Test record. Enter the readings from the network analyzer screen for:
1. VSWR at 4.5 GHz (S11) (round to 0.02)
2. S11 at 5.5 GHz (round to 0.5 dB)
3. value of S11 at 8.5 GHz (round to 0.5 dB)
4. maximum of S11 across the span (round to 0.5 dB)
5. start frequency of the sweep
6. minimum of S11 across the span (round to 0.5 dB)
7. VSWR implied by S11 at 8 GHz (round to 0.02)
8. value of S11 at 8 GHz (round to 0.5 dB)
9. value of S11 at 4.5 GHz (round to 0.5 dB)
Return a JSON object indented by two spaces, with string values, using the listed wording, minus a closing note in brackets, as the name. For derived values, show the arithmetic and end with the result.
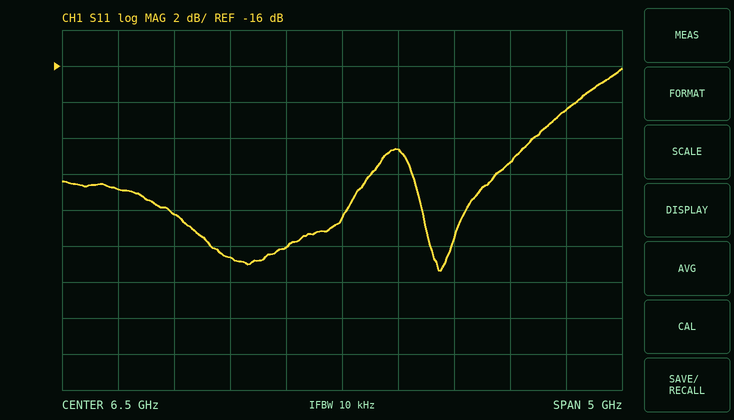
{
  "VSWR at 4.5 GHz (S11)": "|Γ| = 10^(-23/20) = 0.0708; VSWR = (1 + 0.0708)/(1 − 0.0708) ≈ 1.15, so 1.16 to the nearest 0.02",
  "S11 at 5.5 GHz": "-26.5 dB",
  "value of S11 at 8.5 GHz": "-18.5 dB",
  "maximum of S11 across the span": "-16.0 dB",
  "start frequency of the sweep": "4 GHz",
  "minimum of S11 across the span": "-27.5 dB",
  "VSWR implied by S11 at 8 GHz": "|Γ| = 10^(-21.5/20) = 0.0841; VSWR = (1 + 0.0841)/(1 − 0.0841) ≈ 1.18",
  "value of S11 at 8 GHz": "-21.5 dB",
  "value of S11 at 4.5 GHz": "-23.0 dB"
}
